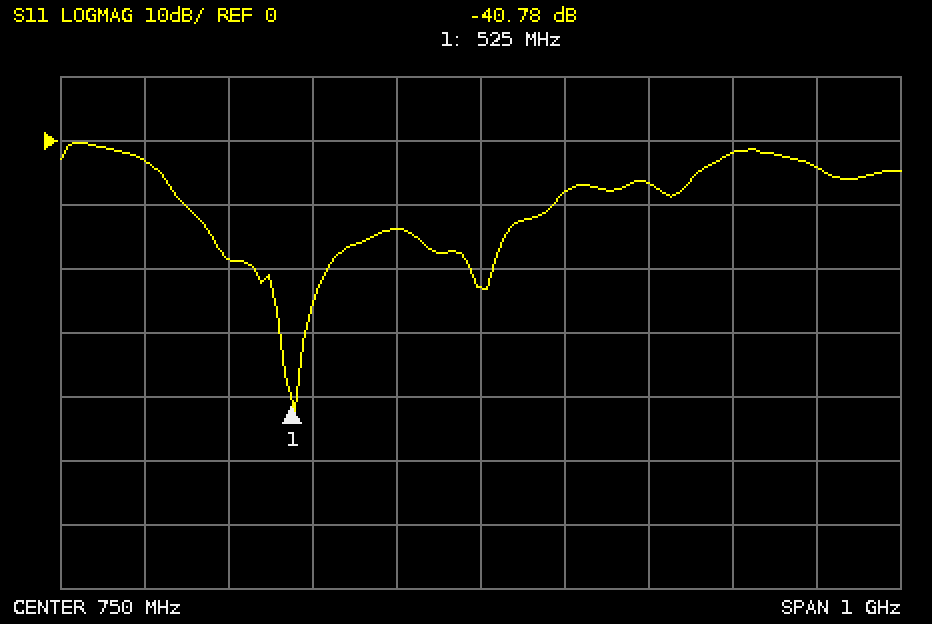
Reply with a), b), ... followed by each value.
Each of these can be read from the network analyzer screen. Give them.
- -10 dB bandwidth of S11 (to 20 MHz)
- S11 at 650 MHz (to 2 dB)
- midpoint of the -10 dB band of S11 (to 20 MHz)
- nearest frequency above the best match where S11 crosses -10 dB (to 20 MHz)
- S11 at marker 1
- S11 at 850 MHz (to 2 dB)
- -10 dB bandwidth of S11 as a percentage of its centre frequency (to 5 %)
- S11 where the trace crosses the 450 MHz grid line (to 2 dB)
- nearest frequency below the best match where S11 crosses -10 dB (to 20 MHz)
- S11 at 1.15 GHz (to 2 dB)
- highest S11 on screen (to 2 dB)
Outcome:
a) 440 MHz
b) -14 dB
c) 620 MHz
d) 840 MHz
e) -40.78 dB
f) -8 dB
g) 70 %
h) -18 dB
i) 400 MHz
j) -4 dB
k) 0 dB
